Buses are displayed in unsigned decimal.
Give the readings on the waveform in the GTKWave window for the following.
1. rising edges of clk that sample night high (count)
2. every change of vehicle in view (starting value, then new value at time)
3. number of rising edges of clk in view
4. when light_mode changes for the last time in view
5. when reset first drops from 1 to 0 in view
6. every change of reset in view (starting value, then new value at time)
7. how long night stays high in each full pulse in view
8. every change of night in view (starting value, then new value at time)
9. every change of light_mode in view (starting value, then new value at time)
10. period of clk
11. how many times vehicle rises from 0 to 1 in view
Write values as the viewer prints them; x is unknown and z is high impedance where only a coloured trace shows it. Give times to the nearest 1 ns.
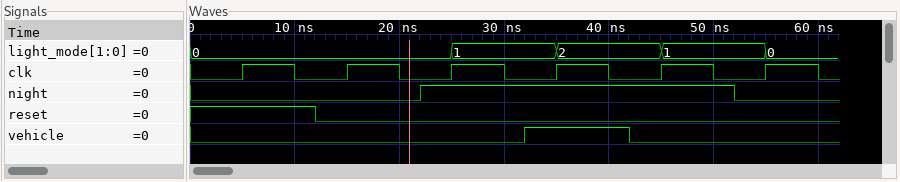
3
0, 1 at 32 ns, 0 at 42 ns
6
55 ns
12 ns
1, 0 at 12 ns
30 ns
0, 1 at 22 ns, 0 at 52 ns
0, 1 at 25 ns, 2 at 35 ns, 1 at 45 ns, 0 at 55 ns
10 ns
1
